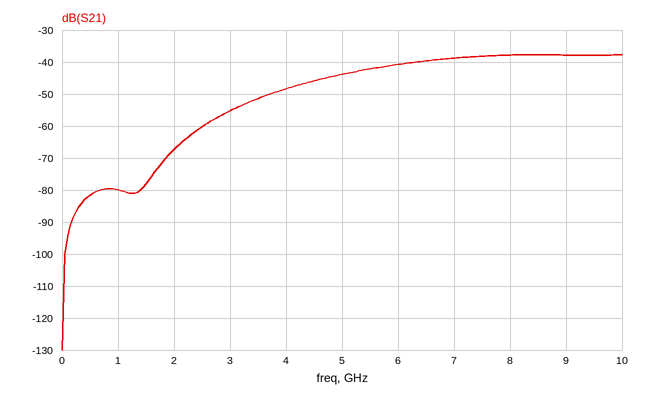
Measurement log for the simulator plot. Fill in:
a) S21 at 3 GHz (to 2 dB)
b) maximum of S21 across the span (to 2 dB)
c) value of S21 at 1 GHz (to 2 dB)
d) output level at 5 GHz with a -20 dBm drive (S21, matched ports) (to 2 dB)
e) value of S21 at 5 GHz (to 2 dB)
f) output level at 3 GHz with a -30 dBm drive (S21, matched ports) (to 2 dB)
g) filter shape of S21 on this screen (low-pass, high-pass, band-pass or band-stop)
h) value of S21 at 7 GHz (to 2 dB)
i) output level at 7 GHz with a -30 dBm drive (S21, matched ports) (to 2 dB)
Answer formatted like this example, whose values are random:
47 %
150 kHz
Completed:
-56 dB
-38 dB
-80 dB
-64 dBm
-44 dB
-86 dBm
high-pass
-38 dB
-68 dBm
